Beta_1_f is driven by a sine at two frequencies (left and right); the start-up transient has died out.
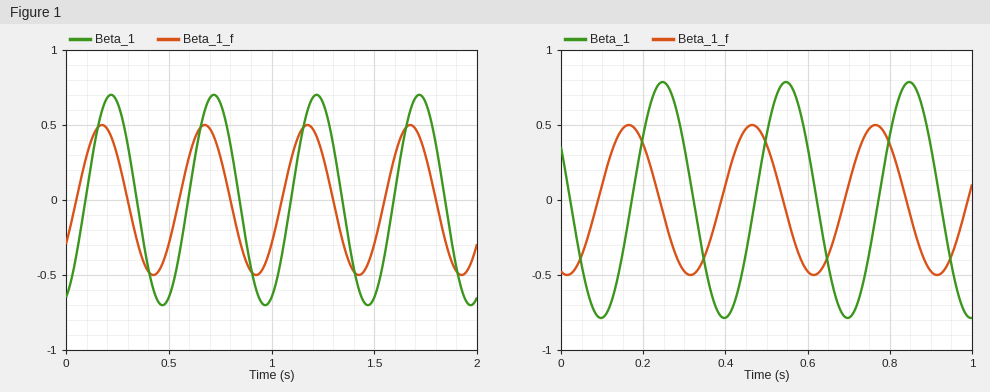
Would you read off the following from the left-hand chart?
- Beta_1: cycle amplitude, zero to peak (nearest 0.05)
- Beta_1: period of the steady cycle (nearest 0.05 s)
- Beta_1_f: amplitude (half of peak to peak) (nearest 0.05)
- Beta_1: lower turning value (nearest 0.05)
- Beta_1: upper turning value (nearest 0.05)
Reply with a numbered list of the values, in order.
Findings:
1. 0.70
2. 0.50 s
3. 0.50
4. -0.70
5. 0.70
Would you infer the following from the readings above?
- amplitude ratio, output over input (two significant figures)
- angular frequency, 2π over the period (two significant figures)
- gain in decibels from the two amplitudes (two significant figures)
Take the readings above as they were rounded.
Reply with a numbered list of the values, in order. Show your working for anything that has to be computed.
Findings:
1. 0.7 / 0.5 = 1.4
2. 2π / 0.5 = 13 rad/s
3. 20 log10(0.7 / 0.5) = 2.9 dB
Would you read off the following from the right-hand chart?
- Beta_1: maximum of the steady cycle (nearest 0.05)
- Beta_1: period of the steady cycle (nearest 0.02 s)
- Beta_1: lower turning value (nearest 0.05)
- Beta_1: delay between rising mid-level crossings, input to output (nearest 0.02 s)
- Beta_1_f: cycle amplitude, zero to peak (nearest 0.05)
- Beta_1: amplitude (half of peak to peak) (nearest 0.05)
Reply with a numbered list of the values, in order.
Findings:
1. 0.80
2. 0.30 s
3. -0.80
4. 0.08 s
5. 0.50
6. 0.80
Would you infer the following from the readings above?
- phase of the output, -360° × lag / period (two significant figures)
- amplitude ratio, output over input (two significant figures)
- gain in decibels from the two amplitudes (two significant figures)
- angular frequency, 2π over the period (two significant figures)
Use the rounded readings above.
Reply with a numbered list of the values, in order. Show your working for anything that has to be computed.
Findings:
1. -360 × 0.08 / 0.3 = -96°
2. 0.8 / 0.5 = 1.6
3. 20 log10(0.8 / 0.5) = 4.1 dB
4. 2π / 0.3 = 21 rad/s
